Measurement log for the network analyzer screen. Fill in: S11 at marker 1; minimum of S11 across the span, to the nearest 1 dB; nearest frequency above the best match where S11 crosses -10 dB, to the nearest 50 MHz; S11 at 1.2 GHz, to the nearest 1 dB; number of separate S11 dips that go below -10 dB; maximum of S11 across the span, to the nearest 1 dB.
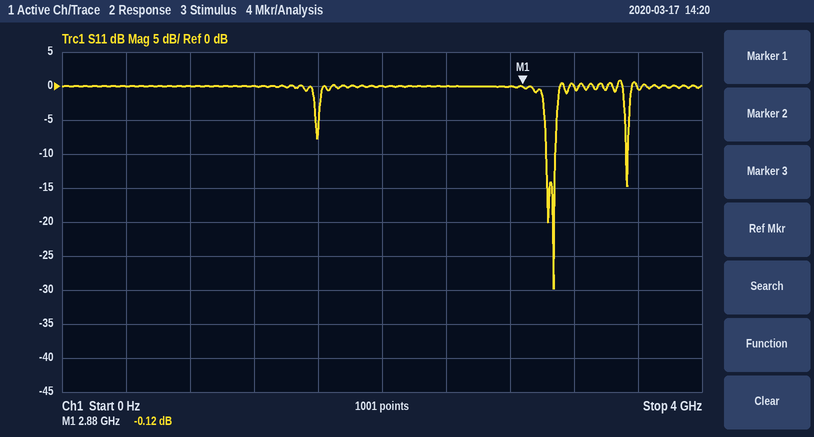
-0.12 dB
-30 dB
3.10 GHz
0 dB
3
1 dB
